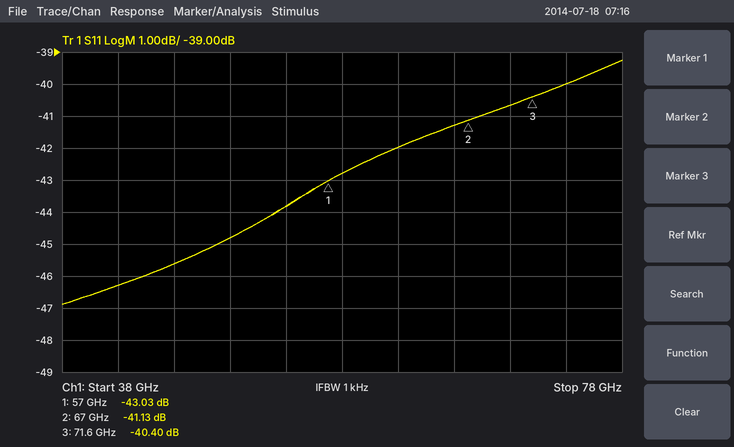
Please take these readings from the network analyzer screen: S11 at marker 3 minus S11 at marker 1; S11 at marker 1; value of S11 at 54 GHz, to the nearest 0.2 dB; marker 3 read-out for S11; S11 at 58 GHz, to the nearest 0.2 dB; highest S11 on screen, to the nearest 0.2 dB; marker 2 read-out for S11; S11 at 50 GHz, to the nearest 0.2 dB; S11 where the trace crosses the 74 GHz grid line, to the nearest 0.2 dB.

2.63 dB
-43.03 dB
-43.8 dB
-40.40 dB
-42.8 dB
-39.2 dB
-41.13 dB
-44.8 dB
-40.0 dB
